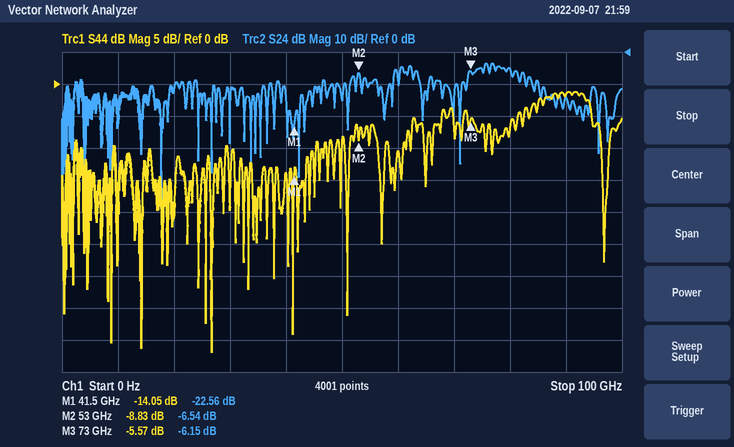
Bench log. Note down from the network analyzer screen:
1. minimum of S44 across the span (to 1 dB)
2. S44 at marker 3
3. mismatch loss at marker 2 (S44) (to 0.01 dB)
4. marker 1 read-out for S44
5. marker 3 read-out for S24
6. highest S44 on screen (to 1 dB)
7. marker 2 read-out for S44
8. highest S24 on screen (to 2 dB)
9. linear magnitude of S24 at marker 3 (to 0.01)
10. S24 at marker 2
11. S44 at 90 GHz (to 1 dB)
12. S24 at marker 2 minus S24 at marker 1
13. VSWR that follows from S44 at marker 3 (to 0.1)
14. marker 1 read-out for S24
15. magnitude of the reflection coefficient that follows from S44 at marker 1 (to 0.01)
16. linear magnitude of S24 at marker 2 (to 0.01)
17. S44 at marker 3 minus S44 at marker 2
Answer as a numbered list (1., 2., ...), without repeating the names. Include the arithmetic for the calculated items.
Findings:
1. -42 dB
2. -5.57 dB
3. −10 log10(1 − 10^(-8.83/10)) ≈ 0.61 dB
4. -14.05 dB
5. -6.15 dB
6. -1 dB
7. -8.83 dB
8. -4 dB
9. 10^(-6.15/20) ≈ 0.49
10. -6.54 dB
11. -2 dB
12. -6.54 − (-22.56) = 16.02 dB
13. (1 + 0.5266)/(1 − 0.5266) ≈ 3.2
14. -22.56 dB
15. 10^(-14.05/20) ≈ 0.20
16. 10^(-6.54/20) ≈ 0.47
17. -5.57 − (-8.83) = 3.26 dB
